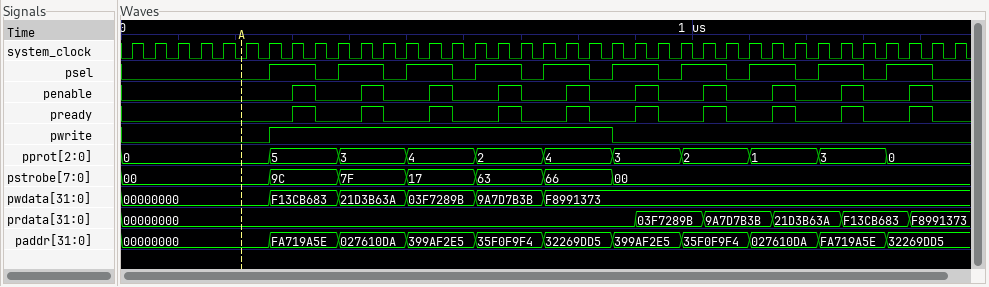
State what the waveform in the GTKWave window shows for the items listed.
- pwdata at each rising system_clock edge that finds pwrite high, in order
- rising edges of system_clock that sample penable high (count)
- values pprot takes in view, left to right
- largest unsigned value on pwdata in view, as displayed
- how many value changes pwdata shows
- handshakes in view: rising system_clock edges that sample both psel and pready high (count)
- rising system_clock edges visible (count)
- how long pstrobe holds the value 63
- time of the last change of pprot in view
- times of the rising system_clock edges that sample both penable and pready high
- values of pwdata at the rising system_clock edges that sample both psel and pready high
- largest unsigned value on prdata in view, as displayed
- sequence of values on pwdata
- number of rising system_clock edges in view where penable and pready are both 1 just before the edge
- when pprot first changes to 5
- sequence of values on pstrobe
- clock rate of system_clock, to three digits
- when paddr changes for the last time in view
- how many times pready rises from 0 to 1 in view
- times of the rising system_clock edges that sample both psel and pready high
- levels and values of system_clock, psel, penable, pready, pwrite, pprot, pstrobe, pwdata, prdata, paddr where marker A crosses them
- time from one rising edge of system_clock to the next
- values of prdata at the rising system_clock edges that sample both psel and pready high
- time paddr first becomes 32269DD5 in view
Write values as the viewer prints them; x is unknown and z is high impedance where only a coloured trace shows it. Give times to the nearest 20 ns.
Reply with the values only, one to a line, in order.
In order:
F13CB683, F13CB683, F13CB683, 21D3B63A, 21D3B63A, 21D3B63A, 03F7289B, 03F7289B, 03F7289B, 9A7D7B3B, 9A7D7B3B, 9A7D7B3B, F8991373, F8991373, F8991373
10
0, 5, 3, 4, 2, 4, 3, 2, 1, 3, 0
F8991373
5
10
37
120 ns
1340 ns
340 ns, 460 ns, 580 ns, 700 ns, 820 ns, 940 ns, 1060 ns, 1180 ns, 1300 ns, 1420 ns
F13CB683, 21D3B63A, 03F7289B, 9A7D7B3B, F8991373, F8991373, F8991373, F8991373, F8991373, F8991373
F8991373
00000000, F13CB683, 21D3B63A, 03F7289B, 9A7D7B3B, F8991373
10
260 ns
00, 9C, 7F, 17, 63, 66, 00
25.0 MHz
1340 ns
10
340 ns, 460 ns, 580 ns, 700 ns, 820 ns, 940 ns, 1060 ns, 1180 ns, 1300 ns, 1420 ns
system_clock=0, psel=0, penable=0, pready=0, pwrite=0, pprot=0, pstrobe=00, pwdata=00000000, prdata=00000000, paddr=00000000
40 ns
00000000, 00000000, 00000000, 00000000, 00000000, 03F7289B, 9A7D7B3B, 21D3B63A, F13CB683, F8991373
740 ns
